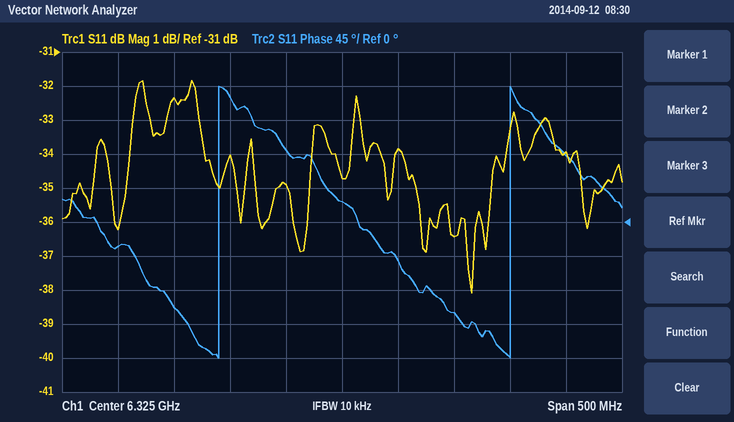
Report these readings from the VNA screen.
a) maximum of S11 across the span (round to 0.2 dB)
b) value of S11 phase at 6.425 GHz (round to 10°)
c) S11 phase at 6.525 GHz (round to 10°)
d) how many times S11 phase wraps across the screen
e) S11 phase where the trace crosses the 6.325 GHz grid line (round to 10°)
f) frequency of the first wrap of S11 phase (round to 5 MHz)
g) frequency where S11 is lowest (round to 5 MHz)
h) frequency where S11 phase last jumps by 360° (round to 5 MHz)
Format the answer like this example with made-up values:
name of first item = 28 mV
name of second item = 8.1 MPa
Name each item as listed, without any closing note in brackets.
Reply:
maximum of S11 across the span = -31.8 dB
value of S11 phase at 6.425 GHz = -120°
S11 phase at 6.525 GHz = 90°
how many times S11 phase wraps across the screen = 2
S11 phase where the trace crosses the 6.325 GHz grid line = 30°
frequency of the first wrap of S11 phase = 6.215 GHz
frequency where S11 is lowest = 6.440 GHz
frequency where S11 phase last jumps by 360° = 6.475 GHz
